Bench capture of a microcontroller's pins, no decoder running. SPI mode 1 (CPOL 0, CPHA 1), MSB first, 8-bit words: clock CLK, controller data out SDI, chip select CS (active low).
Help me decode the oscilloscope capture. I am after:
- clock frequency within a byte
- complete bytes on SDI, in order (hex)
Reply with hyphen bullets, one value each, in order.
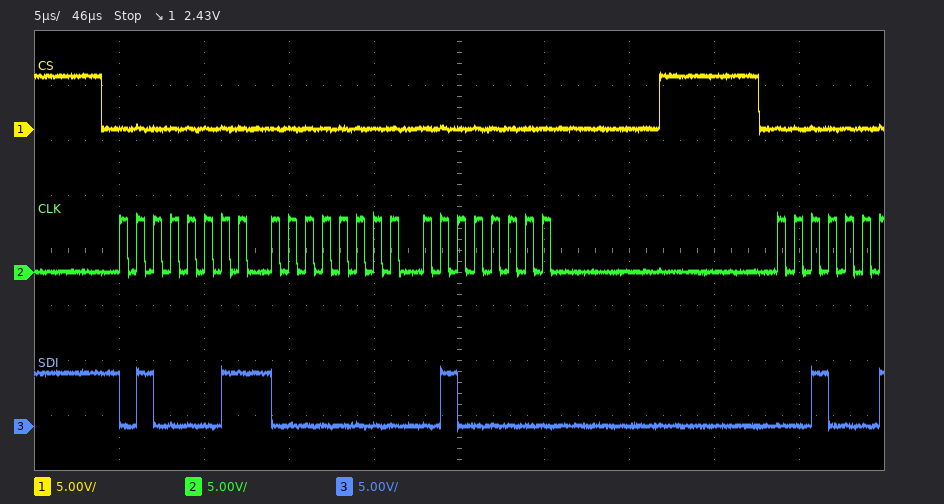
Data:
- 1 MHz
- 43 00 40
